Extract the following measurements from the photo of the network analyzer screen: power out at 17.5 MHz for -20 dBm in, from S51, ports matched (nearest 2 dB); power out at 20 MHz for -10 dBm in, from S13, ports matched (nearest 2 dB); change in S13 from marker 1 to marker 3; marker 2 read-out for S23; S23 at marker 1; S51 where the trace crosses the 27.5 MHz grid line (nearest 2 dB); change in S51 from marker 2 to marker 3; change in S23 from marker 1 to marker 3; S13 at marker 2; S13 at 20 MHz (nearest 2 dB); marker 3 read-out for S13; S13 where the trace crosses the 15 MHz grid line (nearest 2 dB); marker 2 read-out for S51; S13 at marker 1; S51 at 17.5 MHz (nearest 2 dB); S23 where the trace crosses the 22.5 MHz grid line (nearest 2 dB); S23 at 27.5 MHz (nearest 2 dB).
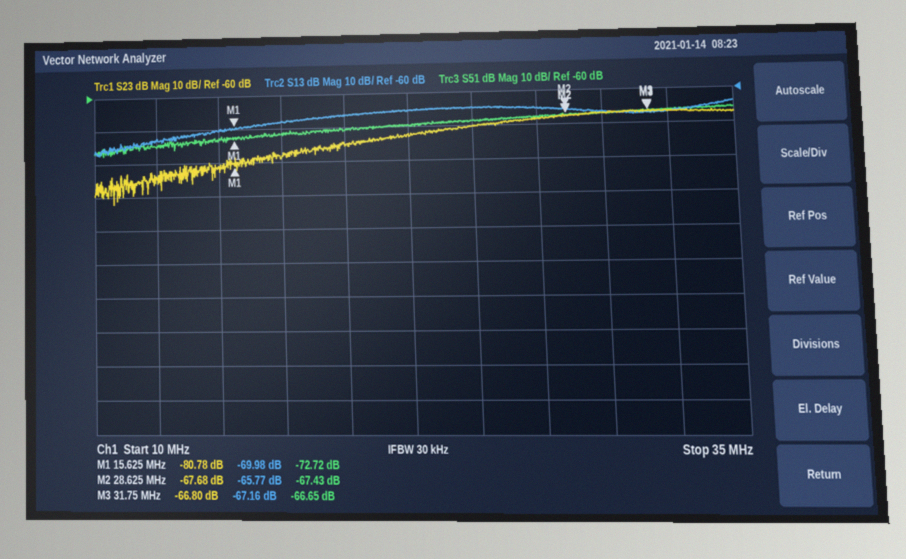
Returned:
-92 dBm
-76 dBm
2.82 dB
-67.68 dB
-80.78 dB
-68 dB
0.78 dB
13.98 dB
-65.77 dB
-66 dB
-67.16 dB
-70 dB
-67.43 dB
-69.98 dB
-72 dB
-72 dB
-68 dB
